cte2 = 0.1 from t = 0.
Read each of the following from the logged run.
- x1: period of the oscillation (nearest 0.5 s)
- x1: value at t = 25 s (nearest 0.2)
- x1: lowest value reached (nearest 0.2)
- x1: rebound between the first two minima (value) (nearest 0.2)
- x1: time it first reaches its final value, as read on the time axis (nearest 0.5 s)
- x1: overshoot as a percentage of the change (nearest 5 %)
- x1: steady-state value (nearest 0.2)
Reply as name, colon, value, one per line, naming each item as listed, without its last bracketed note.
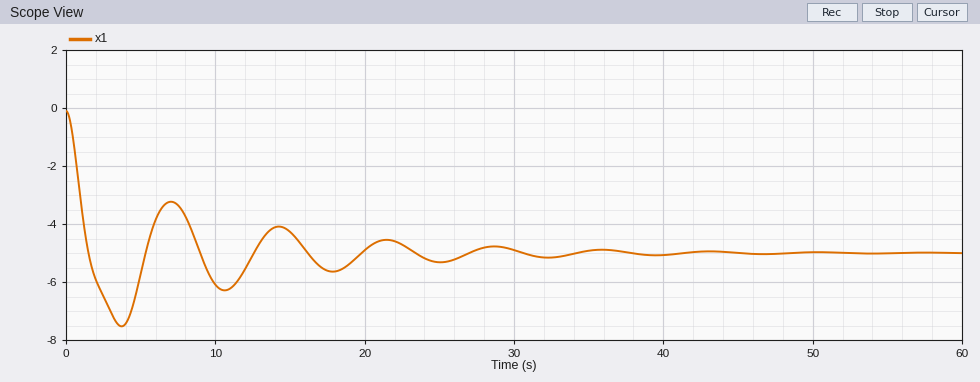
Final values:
x1: period of the oscillation: 7.0 s
x1: value at t = 25 s: -5.4
x1: lowest value reached: -7.6
x1: rebound between the first two minima (value): -3.2
x1: time it first reaches its final value, as read on the time axis: 1.5 s
x1: overshoot as a percentage of the change: 50 %
x1: steady-state value: -5.0
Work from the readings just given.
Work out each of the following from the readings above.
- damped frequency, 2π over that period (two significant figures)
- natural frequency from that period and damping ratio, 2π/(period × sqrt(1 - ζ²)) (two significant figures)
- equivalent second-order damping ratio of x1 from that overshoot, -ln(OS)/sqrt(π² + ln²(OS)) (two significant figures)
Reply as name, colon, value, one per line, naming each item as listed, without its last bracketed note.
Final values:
damped frequency, 2π over that period: 0.90 rad/s
natural frequency from that period and damping ratio, 2π/(period × sqrt(1 - ζ²)): 0.92 rad/s
equivalent second-order damping ratio of x1 from that overshoot, -ln(OS)/sqrt(π² + ln²(OS)): 0.22
